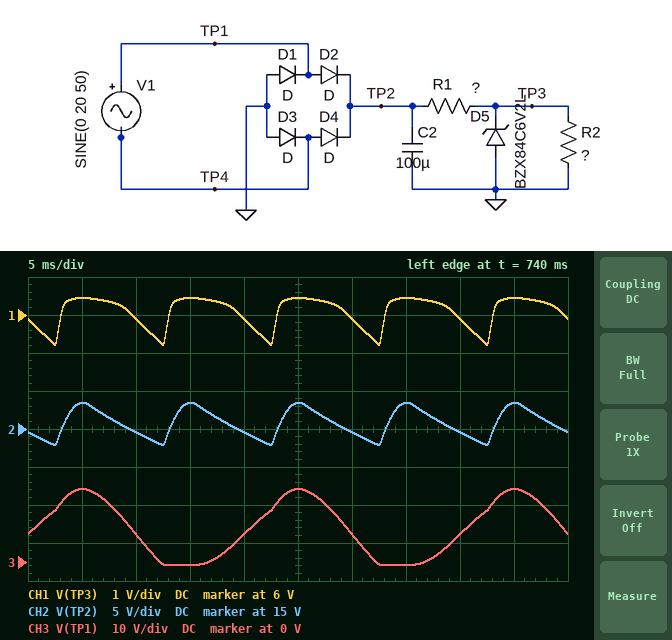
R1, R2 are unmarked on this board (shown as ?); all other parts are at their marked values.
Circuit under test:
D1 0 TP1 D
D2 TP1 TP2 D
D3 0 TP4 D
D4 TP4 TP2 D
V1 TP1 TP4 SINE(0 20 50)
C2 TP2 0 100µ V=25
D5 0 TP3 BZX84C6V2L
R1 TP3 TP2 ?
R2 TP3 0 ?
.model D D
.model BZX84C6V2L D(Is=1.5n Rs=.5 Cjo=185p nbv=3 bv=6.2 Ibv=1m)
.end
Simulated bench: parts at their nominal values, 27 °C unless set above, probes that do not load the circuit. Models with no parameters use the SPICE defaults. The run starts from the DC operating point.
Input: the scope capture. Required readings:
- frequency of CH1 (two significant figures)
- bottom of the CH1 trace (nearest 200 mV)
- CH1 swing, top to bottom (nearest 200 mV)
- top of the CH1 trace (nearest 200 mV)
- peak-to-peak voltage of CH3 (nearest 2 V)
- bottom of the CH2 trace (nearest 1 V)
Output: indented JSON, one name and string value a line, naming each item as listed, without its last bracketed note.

{
  "frequency of CH1": "100 Hz",
  "bottom of the CH1 trace": "5.2 V",
  "CH1 swing, top to bottom": "1.2 V",
  "top of the CH1 trace": "6.4 V",
  "peak-to-peak voltage of CH3": "20 V",
  "bottom of the CH2 trace": "13 V"
}
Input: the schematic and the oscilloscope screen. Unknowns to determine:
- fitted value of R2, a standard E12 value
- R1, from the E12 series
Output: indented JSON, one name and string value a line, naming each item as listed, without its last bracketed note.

{
  "fitted value of R2, a standard E12 value": "82 Ω",
  "R1, from the E12 series": "120 Ω"
}
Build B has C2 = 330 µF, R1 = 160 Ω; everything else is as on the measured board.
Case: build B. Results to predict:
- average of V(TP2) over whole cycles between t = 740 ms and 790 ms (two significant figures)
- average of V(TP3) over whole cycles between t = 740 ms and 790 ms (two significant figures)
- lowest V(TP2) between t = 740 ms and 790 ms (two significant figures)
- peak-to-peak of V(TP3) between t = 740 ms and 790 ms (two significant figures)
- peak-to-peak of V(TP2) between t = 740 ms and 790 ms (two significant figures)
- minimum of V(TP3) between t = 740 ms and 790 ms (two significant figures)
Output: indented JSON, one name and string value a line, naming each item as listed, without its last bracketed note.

{
  "average of V(TP2) over whole cycles between t = 740 ms and 790 ms": "18 V",
  "average of V(TP3) over whole cycles between t = 740 ms and 790 ms": "5.9 V",
  "lowest V(TP2) between t = 740 ms and 790 ms": "17 V",
  "peak-to-peak of V(TP3) between t = 740 ms and 790 ms": "570 mV",
  "peak-to-peak of V(TP2) between t = 740 ms and 790 ms": "1.8 V",
  "minimum of V(TP3) between t = 740 ms and 790 ms": "5.6 V"
}
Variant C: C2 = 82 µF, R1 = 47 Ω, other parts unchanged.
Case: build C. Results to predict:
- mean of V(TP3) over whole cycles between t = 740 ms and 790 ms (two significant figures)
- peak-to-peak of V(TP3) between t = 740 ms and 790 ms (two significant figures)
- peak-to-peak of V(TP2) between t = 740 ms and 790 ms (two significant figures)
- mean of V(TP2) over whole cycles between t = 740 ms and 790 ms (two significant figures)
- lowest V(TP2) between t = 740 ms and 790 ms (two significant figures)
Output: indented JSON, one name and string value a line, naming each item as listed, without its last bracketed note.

{
  "mean of V(TP3) over whole cycles between t = 740 ms and 790 ms": "6.5 V",
  "peak-to-peak of V(TP3) between t = 740 ms and 790 ms": "1.0 V",
  "peak-to-peak of V(TP2) between t = 740 ms and 790 ms": "9.5 V",
  "mean of V(TP2) over whole cycles between t = 740 ms and 790 ms": "14 V",
  "lowest V(TP2) between t = 740 ms and 790 ms": "8.9 V"
}
